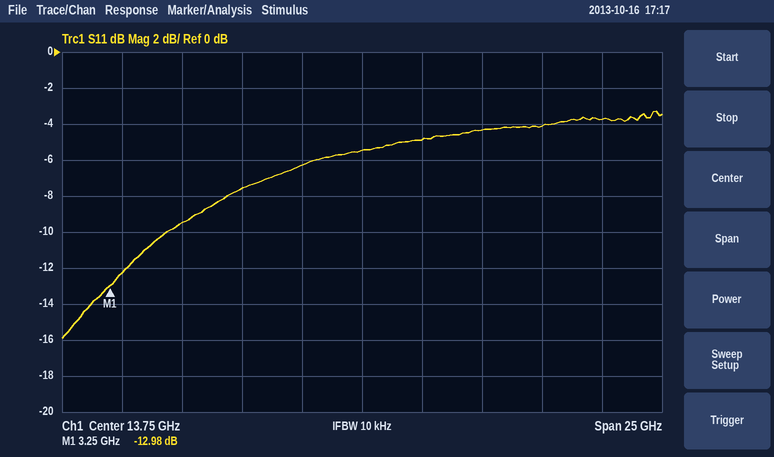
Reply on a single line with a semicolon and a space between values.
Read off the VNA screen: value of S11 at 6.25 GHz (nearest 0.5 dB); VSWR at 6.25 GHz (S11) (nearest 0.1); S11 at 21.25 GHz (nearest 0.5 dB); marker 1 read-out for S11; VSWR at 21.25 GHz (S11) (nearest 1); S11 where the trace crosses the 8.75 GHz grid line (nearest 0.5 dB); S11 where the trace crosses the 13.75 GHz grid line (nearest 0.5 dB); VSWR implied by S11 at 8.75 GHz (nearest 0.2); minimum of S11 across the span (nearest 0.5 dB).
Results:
-9.5 dB; 2.0; -4.0 dB; -12.98 dB; 4; -7.5 dB; -5.5 dB; 2.4; -16.0 dB
